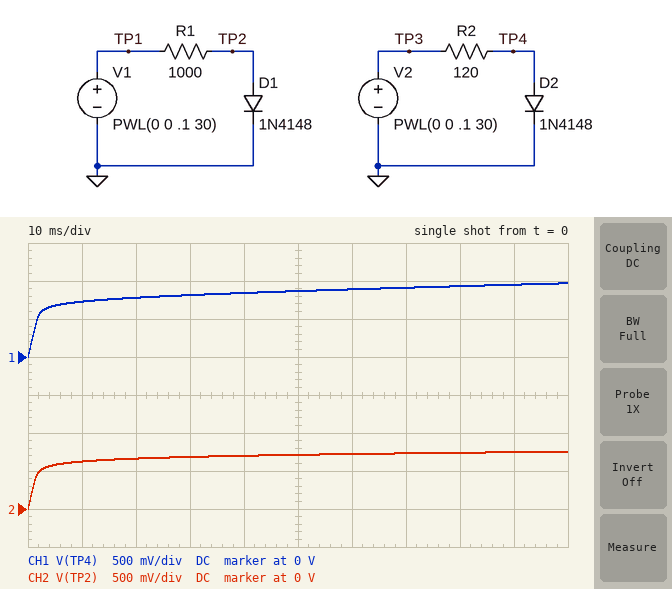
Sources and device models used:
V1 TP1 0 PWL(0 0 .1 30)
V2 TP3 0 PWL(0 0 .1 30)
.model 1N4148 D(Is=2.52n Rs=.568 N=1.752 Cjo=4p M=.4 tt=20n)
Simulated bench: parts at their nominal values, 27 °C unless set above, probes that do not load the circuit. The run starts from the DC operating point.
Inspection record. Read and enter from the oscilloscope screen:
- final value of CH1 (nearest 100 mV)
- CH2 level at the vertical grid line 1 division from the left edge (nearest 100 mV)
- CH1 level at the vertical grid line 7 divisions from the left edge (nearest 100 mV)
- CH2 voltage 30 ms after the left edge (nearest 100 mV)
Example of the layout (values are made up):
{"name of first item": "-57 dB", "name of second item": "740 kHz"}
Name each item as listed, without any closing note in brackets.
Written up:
{"final value of CH1": "1.0 V", "CH2 level at the vertical grid line 1 division from the left edge": "600 mV", "CH1 level at the vertical grid line 7 divisions from the left edge": "900 mV", "CH2 voltage 30 ms after the left edge": "700 mV"}
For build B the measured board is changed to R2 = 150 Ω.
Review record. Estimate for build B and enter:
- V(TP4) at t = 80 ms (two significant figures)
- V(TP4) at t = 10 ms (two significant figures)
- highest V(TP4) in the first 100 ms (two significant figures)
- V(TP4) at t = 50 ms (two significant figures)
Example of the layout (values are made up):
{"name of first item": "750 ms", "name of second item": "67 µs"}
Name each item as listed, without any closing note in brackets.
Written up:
{"V(TP4) at t = 80 ms": "900 mV", "V(TP4) at t = 10 ms": "720 mV", "highest V(TP4) in the first 100 ms": "930 mV", "V(TP4) at t = 50 ms": "840 mV"}
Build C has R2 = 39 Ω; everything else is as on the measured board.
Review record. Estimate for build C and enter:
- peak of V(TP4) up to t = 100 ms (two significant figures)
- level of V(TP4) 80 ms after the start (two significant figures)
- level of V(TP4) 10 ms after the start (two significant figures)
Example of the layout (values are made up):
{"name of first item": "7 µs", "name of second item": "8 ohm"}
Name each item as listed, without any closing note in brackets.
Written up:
{"peak of V(TP4) up to t = 100 ms": "1.3 V", "level of V(TP4) 80 ms after the start": "1.2 V", "level of V(TP4) 10 ms after the start": "800 mV"}
